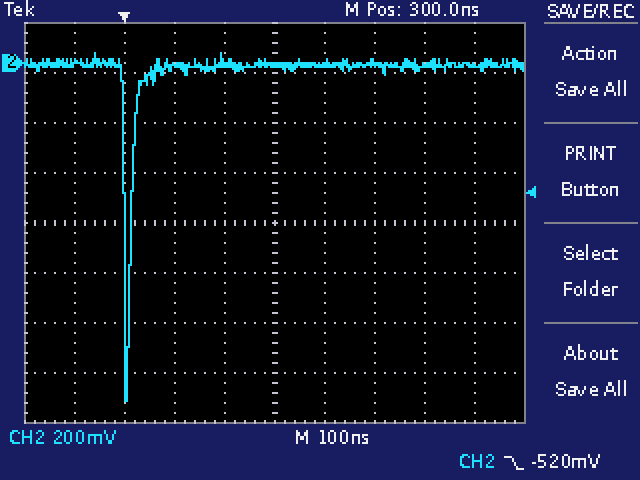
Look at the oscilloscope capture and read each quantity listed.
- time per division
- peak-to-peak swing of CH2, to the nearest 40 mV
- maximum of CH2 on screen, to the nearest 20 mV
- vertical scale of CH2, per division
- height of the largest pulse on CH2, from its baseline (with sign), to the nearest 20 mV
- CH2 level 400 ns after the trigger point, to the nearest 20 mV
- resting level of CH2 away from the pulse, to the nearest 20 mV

100 ns
1.40 V
40 mV
200 mV
-1.34 V
0 mV
0 mV
